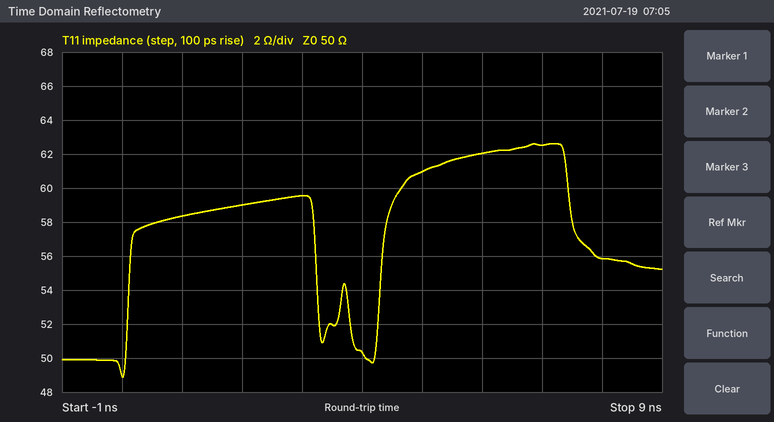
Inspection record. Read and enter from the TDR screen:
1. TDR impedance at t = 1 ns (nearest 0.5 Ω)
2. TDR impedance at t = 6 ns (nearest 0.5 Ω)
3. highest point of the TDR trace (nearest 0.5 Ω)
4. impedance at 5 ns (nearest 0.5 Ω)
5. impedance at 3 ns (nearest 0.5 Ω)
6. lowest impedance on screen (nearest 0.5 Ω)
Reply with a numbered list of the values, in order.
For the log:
1. 58.5 Ω
2. 62.0 Ω
3. 62.5 Ω
4. 61.0 Ω
5. 59.5 Ω
6. 49.0 Ω
